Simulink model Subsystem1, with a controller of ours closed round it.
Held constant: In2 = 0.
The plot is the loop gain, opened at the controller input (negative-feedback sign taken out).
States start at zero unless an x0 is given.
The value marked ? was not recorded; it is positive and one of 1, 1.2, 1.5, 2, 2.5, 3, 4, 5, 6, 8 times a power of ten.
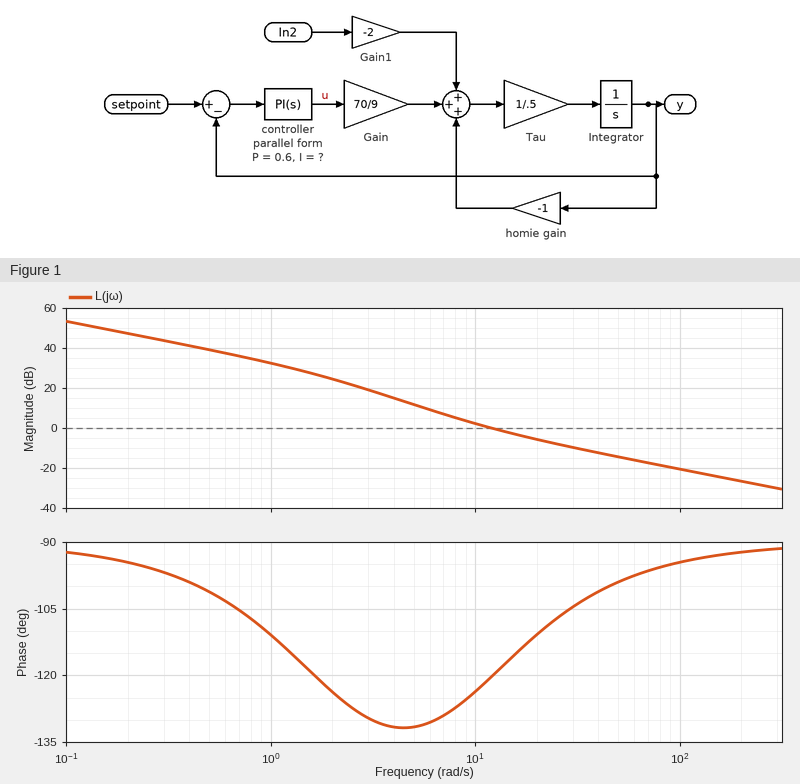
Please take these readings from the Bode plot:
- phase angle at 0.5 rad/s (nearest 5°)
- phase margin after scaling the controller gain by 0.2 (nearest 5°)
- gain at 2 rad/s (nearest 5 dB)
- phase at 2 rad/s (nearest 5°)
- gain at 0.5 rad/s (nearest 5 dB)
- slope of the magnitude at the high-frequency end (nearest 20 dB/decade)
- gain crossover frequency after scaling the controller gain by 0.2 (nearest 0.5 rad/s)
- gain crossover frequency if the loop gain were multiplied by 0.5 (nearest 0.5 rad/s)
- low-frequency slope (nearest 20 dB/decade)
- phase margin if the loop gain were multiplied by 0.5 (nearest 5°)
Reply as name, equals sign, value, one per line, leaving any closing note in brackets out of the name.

phase angle at 0.5 rad/s = -100°
phase margin after scaling the controller gain by 0.2 = 50°
gain at 2 rad/s = 25 dB
phase at 2 rad/s = -125°
gain at 0.5 rad/s = 40 dB
slope of the magnitude at the high-frequency end = -20 dB/decade
gain crossover frequency after scaling the controller gain by 0.2 = 4.5 rad/s
gain crossover frequency if the loop gain were multiplied by 0.5 = 7.5 rad/s
low-frequency slope = -20 dB/decade
phase margin if the loop gain were multiplied by 0.5 = 50°
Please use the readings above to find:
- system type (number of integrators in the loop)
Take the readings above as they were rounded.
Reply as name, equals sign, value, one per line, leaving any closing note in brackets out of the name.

system type = 1
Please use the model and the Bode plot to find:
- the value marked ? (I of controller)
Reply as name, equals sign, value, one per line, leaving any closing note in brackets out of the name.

the value marked ? = 6
